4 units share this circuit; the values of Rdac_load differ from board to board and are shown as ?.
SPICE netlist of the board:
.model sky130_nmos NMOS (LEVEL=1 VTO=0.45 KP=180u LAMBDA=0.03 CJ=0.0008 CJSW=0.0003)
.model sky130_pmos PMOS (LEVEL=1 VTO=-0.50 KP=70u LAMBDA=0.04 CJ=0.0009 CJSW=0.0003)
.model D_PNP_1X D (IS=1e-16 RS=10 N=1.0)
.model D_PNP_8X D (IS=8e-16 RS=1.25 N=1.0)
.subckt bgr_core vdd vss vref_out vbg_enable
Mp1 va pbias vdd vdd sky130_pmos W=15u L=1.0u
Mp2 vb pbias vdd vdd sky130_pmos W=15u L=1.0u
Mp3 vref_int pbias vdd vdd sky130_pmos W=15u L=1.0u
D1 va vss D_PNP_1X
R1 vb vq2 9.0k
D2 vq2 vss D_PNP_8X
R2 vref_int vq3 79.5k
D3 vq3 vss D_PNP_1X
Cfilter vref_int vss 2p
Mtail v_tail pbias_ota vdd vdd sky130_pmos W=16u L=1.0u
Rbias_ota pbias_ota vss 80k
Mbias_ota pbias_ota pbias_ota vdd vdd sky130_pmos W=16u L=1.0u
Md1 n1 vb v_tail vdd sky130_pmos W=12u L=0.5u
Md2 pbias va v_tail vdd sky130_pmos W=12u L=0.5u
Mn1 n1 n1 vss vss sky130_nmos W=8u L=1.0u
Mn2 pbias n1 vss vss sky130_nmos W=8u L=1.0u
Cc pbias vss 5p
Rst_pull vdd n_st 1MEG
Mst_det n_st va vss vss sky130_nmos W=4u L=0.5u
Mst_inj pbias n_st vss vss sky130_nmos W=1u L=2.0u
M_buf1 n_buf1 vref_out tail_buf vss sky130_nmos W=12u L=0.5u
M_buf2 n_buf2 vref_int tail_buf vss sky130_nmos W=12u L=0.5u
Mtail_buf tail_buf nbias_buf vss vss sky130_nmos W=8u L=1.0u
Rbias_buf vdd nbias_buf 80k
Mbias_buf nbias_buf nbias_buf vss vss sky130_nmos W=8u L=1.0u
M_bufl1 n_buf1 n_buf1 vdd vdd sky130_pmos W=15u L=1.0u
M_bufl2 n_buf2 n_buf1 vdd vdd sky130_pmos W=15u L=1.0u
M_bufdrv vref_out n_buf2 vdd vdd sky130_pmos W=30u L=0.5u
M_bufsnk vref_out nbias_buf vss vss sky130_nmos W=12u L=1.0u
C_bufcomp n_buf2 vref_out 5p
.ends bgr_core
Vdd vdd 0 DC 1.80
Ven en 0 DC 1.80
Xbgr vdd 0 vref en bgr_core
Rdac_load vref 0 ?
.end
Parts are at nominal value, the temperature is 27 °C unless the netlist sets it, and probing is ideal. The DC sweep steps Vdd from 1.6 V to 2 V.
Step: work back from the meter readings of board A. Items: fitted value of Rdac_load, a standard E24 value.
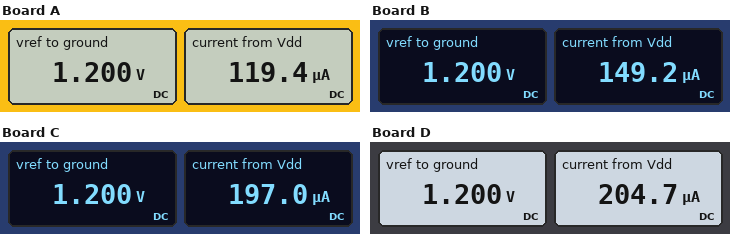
82 kΩ
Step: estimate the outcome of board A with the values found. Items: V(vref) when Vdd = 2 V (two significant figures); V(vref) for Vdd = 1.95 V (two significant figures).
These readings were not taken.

1.8 V
1.7 V
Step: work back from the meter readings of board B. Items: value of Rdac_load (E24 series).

27 kΩ
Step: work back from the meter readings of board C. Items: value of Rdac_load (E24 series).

13 kΩ
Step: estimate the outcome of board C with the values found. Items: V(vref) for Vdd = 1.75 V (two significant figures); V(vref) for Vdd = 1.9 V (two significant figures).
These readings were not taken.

1.1 V
1.5 V
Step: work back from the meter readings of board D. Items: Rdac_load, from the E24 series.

12 kΩ
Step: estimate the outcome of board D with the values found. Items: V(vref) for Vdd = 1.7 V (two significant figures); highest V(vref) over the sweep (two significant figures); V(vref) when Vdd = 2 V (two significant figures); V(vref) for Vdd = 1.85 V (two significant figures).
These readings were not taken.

1.1 V
1.7 V
1.7 V
1.3 V
